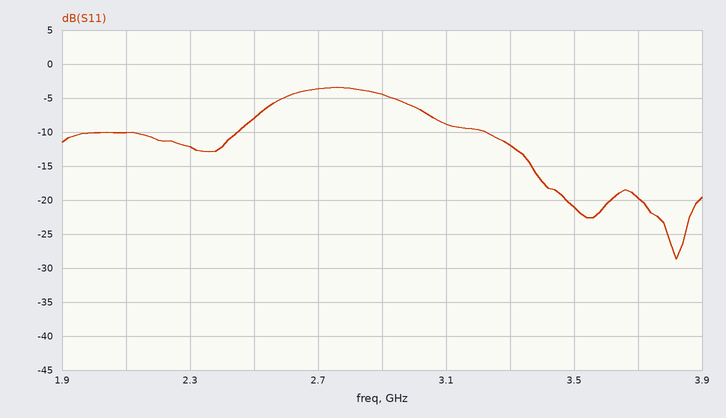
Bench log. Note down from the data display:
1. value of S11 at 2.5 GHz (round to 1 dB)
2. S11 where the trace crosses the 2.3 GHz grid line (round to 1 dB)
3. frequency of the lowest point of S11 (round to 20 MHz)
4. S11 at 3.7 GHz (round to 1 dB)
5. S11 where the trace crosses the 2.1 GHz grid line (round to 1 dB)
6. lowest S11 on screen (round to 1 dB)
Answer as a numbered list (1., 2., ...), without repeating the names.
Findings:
1. -8 dB
2. -12 dB
3. 3.82 GHz
4. -20 dB
5. -10 dB
6. -29 dB
